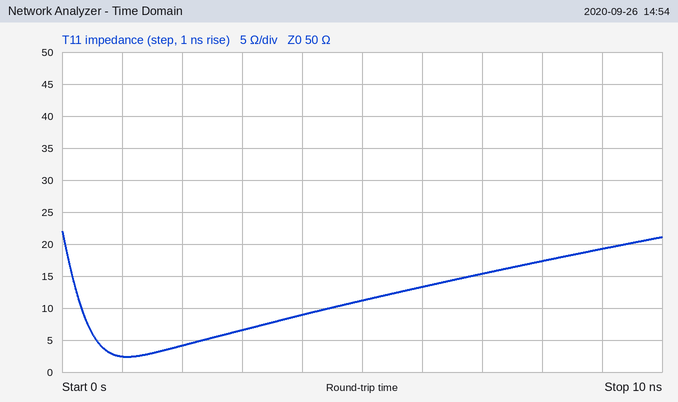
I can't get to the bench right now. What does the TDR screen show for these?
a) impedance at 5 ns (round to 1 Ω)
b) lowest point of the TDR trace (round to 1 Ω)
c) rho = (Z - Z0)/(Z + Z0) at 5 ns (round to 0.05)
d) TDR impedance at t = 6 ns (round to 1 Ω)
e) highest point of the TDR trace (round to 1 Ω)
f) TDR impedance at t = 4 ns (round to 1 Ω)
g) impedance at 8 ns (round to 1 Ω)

11 Ω
2 Ω
-0.65
13 Ω
22 Ω
9 Ω
17 Ω
